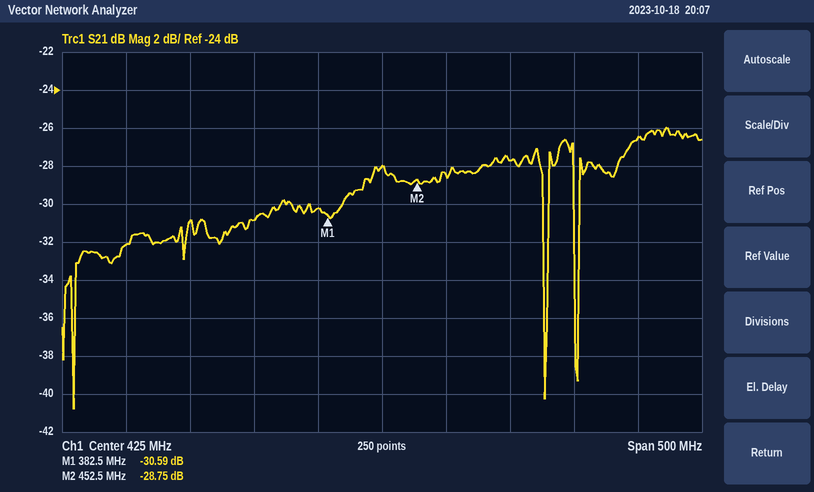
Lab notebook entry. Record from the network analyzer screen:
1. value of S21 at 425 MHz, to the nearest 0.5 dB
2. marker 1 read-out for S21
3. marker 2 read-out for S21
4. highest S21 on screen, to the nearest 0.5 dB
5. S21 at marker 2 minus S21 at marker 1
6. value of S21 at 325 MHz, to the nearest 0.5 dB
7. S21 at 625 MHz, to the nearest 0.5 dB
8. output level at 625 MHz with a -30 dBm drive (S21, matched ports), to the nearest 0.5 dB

-28.0 dB
-30.59 dB
-28.75 dB
-26.0 dB
1.84 dB
-31.0 dB
-26.5 dB
-56.5 dBm
